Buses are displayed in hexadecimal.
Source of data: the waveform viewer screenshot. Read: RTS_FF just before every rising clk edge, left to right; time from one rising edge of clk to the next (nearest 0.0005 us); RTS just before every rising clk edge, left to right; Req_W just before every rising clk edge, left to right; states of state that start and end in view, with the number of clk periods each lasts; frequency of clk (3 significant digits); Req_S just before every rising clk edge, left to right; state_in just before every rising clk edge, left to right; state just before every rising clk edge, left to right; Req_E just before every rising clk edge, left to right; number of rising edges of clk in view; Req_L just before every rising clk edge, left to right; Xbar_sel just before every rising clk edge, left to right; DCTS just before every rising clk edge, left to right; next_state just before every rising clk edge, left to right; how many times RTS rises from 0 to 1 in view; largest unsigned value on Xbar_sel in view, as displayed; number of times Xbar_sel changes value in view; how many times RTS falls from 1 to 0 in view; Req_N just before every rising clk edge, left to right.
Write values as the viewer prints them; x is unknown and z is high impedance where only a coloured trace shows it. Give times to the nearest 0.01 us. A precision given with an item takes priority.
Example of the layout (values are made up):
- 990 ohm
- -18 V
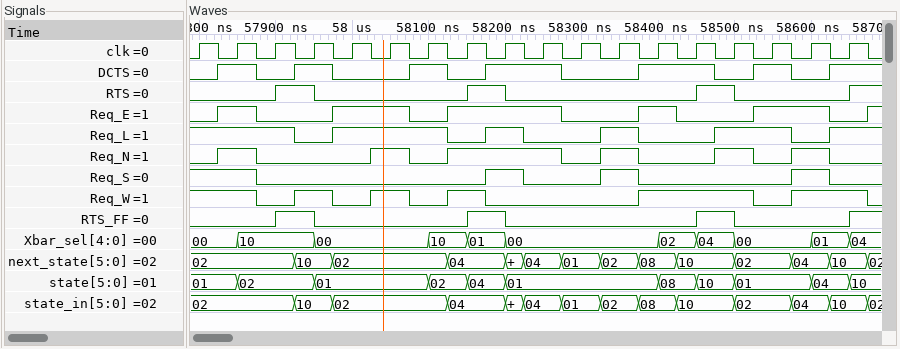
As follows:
- 0 0 0 1 0 0 0 0 1 0 0 0 0 0 1 0 0 0
- 0.05 us
- 0 0 0 1 0 0 0 0 1 0 0 0 0 0 1 0 0 0
- 1 1 0 1 0 1 0 1 0 0 0 0 1 1 1 0 1 1
- 02: 2, 01: 3, 02: 1, 04: 1, 01: 4, 08: 1, 10: 1, 01: 2, 04: 1
- 20.0 MHz
- 1 1 0 0 0 0 0 0 1 0 0 1 0 0 0 0 1 0
- 02, 02, 02, 10, 02, 02, 02, 04, 04, 04, 01, 02, 08, 10, 10, 02, 04, 10
- 01, 01, 02, 02, 01, 01, 01, 02, 04, 01, 01, 01, 01, 08, 10, 01, 01, 04
- 0 1 0 0 1 1 0 1 1 1 0 0 1 0 0 1 1 0
- 18
- 1 1 1 0 1 1 1 0 1 0 0 1 0 0 1 1 0 1
- 00, 00, 10, 10, 00, 00, 00, 10, 01, 00, 00, 00, 00, 02, 04, 00, 00, 01
- 0 1 0 1 0 0 1 0 1 1 0 0 1 1 0 1 0 1
- 02, 02, 02, 10, 02, 02, 02, 04, 04, 04, 01, 02, 08, 10, 10, 02, 04, 10
- 4
- 10
- 10
- 3
- 0 1 0 0 0 1 0 1 1 1 0 1 0 0 1 0 1 0
